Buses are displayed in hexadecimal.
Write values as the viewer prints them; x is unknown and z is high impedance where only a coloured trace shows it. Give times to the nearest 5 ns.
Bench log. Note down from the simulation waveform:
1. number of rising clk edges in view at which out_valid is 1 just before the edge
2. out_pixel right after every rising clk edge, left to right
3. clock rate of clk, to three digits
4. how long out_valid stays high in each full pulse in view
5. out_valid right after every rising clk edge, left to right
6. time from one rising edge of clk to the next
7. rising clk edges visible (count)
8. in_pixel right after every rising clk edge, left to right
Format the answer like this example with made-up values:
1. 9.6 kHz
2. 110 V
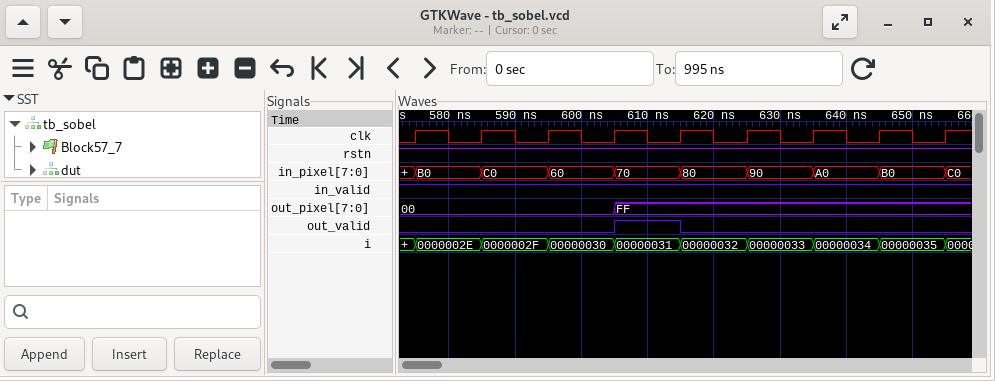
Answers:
1. 1
2. 00, 00, 00, FF, FF, FF, FF, FF, FF
3. 100 MHz
4. 10 ns
5. 0 0 0 1 0 0 0 0 0
6. 10 ns
7. 9
8. B0, C0, 60, 70, 80, 90, A0, B0, C0
